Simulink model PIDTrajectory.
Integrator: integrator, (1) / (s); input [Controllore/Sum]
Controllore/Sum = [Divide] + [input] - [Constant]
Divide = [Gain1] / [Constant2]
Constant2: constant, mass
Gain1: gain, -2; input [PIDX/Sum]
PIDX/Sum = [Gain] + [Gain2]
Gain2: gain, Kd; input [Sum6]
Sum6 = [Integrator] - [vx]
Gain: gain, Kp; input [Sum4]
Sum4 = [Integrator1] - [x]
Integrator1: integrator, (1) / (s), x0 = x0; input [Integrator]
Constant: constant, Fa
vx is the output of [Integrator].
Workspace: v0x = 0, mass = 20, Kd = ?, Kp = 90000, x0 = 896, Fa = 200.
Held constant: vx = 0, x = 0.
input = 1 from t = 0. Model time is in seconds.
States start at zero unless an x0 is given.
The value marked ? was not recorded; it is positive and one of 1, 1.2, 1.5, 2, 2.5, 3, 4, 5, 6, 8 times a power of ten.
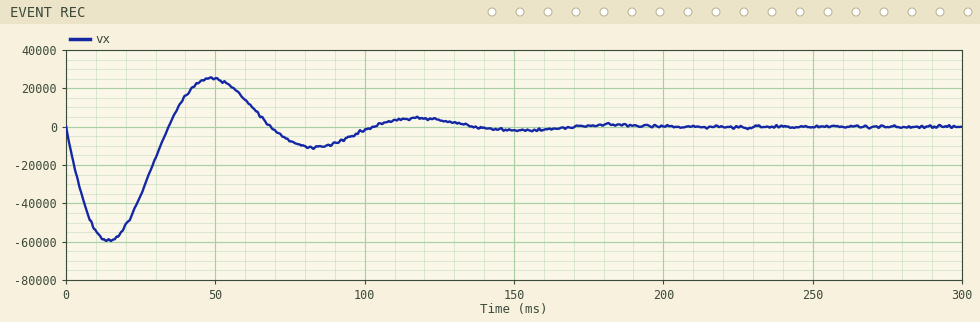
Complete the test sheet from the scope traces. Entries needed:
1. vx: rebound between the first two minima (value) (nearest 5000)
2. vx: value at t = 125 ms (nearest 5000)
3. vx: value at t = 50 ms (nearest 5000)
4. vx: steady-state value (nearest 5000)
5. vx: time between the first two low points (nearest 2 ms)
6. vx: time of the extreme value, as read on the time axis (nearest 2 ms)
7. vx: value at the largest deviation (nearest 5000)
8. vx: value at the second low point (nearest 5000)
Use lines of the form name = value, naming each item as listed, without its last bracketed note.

vx: rebound between the first two minima (value) = 25000
vx: value at t = 125 ms = 5000
vx: value at t = 50 ms = 25000
vx: steady-state value = 0
vx: time between the first two low points = 68 ms
vx: time of the extreme value, as read on the time axis = 14 ms
vx: value at the largest deviation = -60000
vx: value at the second low point = -10000
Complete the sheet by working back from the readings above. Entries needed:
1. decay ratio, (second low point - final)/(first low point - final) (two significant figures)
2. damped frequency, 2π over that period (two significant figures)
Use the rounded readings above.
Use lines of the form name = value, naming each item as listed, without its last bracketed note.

decay ratio, (second low point - final)/(first low point - final) = 0.17
damped frequency, 2π over that period = 0.092 rad/ms
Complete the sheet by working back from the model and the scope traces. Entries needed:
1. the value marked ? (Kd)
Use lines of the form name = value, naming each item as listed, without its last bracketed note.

the value marked ? = 500
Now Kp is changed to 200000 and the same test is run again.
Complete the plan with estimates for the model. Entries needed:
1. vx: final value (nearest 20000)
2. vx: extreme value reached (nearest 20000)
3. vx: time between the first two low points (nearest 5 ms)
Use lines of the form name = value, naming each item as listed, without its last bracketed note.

vx: final value = 0
vx: extreme value reached = -100000
vx: time between the first two low points = 45 ms
